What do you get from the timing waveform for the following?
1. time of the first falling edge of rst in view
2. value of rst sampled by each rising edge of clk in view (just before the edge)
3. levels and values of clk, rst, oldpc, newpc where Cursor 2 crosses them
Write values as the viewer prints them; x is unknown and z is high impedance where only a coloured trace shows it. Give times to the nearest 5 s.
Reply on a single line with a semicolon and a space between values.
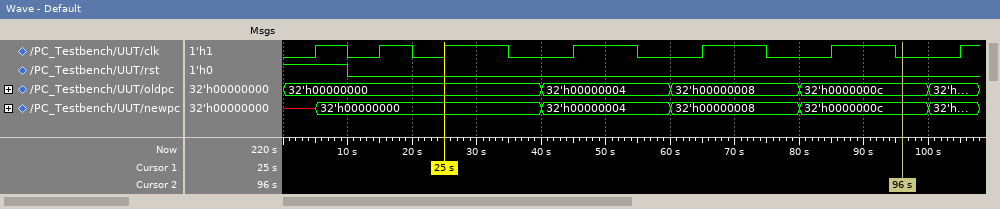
10 s; 1 0 0 0 0 0 0; clk=0, rst=0, oldpc=32'h0000000c, newpc=32'h0000000c
